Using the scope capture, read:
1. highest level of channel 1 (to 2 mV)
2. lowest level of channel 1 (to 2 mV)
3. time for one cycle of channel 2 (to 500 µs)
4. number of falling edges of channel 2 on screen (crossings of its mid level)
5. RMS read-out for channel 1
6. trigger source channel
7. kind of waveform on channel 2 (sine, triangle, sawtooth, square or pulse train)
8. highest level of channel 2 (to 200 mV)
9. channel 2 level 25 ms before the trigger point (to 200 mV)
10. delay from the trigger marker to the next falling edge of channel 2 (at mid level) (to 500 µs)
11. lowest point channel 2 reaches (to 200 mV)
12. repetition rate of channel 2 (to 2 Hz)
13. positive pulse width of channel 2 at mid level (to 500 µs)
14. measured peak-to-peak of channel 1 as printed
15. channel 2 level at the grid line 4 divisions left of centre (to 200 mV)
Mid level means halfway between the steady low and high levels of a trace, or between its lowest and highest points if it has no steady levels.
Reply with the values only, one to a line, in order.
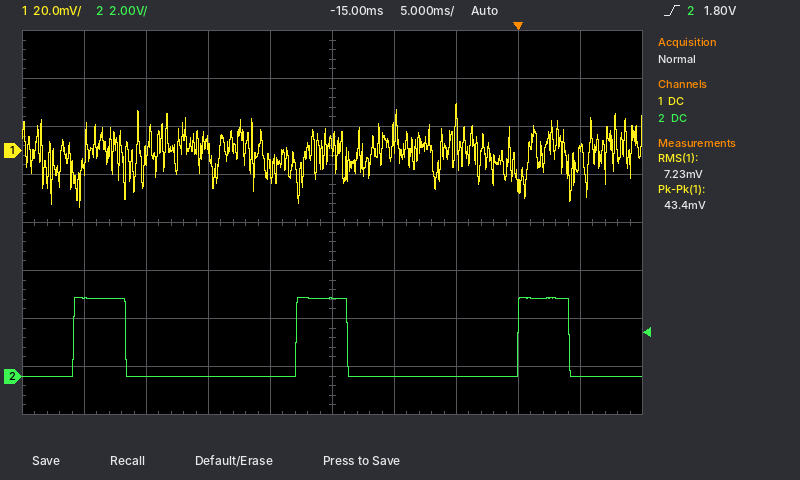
20 mV
-24 mV
18.0 ms
3
7.23 mV
channel 2
pulse train
3.2 V
0.0 V
4.0 ms
0.0 V
56 Hz
4.0 ms
43.4 mV
3.2 V
